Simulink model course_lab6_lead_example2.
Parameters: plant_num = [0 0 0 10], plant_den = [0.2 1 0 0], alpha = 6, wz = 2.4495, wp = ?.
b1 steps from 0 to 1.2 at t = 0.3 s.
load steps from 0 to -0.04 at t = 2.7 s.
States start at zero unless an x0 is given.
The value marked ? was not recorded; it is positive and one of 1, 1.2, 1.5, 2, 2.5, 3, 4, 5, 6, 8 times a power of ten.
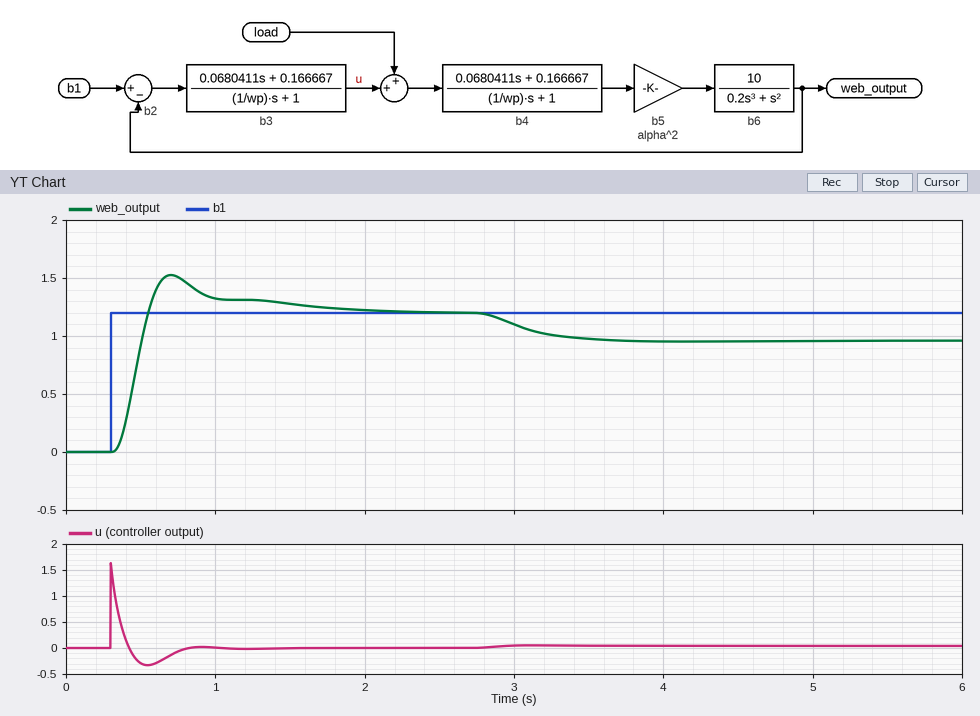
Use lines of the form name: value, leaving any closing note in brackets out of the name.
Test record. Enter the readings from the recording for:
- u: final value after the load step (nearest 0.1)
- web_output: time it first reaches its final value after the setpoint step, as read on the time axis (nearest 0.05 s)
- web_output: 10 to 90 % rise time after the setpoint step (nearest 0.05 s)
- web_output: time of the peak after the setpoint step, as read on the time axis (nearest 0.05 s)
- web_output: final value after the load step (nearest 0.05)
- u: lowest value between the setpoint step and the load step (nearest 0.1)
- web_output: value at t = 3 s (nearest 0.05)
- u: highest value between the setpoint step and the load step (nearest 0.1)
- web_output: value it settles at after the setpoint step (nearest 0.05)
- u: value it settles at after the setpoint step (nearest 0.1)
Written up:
u: final value after the load step: 0.0
web_output: time it first reaches its final value after the setpoint step, as read on the time axis: 0.55 s
web_output: 10 to 90 % rise time after the setpoint step: 0.15 s
web_output: time of the peak after the setpoint step, as read on the time axis: 0.70 s
web_output: final value after the load step: 0.95
u: lowest value between the setpoint step and the load step: -0.3
web_output: value at t = 3 s: 1.10
u: highest value between the setpoint step and the load step: 1.6
web_output: value it settles at after the setpoint step: 1.20
u: value it settles at after the setpoint step: 0.0
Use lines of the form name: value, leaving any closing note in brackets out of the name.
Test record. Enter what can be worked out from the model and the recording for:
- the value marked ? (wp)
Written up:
the value marked ?: 20
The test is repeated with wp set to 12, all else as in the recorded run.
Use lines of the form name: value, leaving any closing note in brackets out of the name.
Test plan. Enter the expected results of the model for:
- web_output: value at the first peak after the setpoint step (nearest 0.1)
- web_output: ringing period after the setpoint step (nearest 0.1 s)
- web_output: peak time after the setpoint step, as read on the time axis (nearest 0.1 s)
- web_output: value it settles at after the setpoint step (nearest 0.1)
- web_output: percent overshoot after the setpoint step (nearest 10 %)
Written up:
web_output: value at the first peak after the setpoint step: 1.8
web_output: ringing period after the setpoint step: 0.9 s
web_output: peak time after the setpoint step, as read on the time axis: 0.8 s
web_output: value it settles at after the setpoint step: 1.2
web_output: percent overshoot after the setpoint step: 50 %
